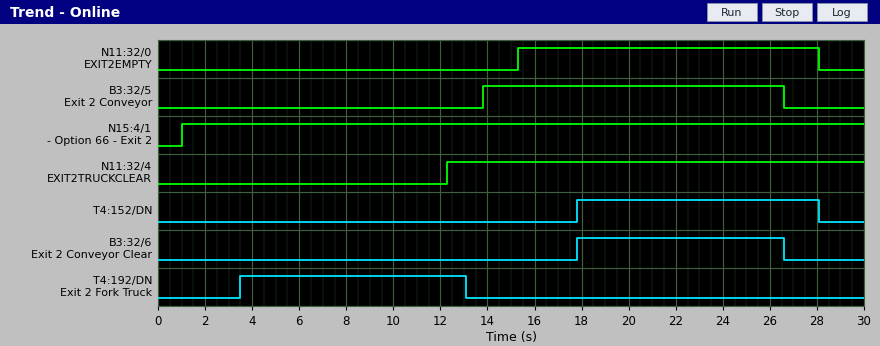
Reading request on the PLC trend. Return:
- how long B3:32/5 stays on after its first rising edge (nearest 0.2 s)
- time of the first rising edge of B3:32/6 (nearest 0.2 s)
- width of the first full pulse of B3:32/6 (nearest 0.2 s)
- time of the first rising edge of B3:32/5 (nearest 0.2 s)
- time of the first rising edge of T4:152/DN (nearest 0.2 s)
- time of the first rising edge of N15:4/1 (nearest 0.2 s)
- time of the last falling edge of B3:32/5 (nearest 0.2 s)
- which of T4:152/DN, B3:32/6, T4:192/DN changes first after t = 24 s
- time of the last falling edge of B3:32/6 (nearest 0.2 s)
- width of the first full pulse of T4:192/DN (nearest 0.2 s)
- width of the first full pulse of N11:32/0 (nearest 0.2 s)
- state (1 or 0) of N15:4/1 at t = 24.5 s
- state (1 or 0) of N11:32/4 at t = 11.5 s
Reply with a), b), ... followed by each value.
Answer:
a) 12.8 s
b) 17.8 s
c) 8.8 s
d) 13.8 s
e) 17.8 s
f) 1.0 s
g) 26.6 s
h) B3:32/6
i) 26.6 s
j) 9.6 s
k) 12.8 s
l) 1
m) 0
